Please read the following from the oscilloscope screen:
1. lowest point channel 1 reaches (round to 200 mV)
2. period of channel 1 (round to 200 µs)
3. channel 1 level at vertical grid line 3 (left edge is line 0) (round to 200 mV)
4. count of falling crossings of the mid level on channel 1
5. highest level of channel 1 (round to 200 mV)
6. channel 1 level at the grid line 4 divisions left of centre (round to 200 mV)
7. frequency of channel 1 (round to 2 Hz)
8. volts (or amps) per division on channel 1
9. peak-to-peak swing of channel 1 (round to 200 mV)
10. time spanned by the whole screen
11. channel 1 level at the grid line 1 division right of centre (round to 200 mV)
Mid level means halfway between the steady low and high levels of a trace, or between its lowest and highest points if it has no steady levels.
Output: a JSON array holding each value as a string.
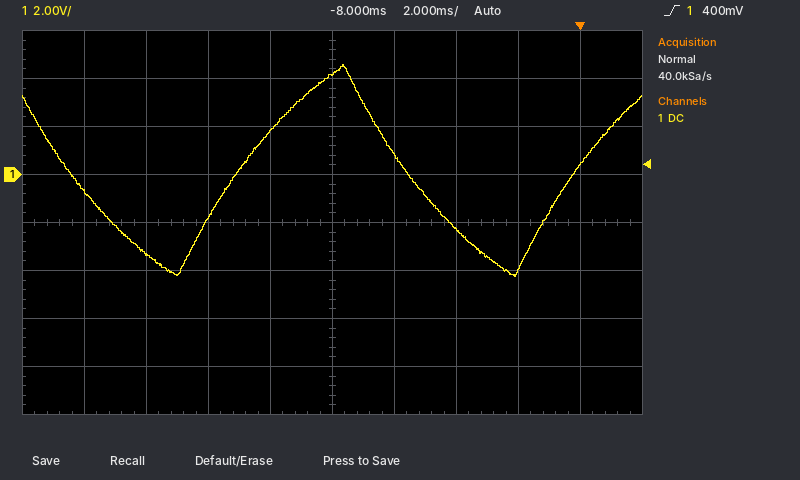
["-4.2 V", "10.8 ms", "-1.8 V", "2", "4.6 V", "-800 mV", "92 Hz", "2 V", "8.8 V", "20 ms", "800 mV"]
